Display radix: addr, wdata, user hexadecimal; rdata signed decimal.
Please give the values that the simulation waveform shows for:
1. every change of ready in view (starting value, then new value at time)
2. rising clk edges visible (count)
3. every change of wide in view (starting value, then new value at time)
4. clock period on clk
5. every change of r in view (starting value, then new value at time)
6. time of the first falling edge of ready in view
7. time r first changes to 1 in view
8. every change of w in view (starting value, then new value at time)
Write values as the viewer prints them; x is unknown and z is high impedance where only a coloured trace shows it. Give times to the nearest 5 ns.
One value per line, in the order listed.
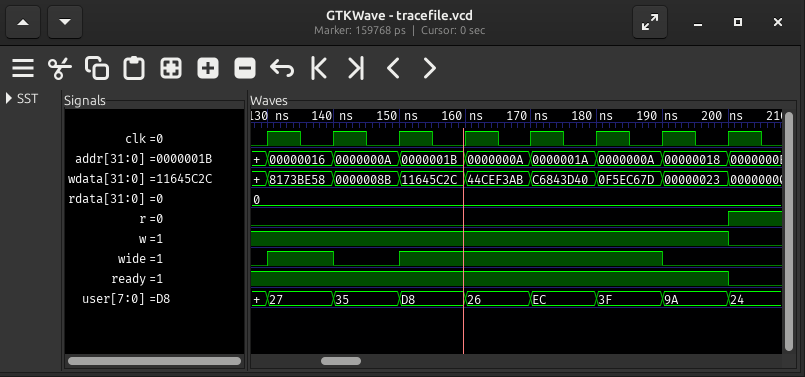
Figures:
1, 0 at 200 ns
8
0, 1 at 130 ns, 0 at 140 ns, 1 at 150 ns, 0 at 190 ns
10 ns
0, 1 at 200 ns
200 ns
200 ns
1, 0 at 200 ns
